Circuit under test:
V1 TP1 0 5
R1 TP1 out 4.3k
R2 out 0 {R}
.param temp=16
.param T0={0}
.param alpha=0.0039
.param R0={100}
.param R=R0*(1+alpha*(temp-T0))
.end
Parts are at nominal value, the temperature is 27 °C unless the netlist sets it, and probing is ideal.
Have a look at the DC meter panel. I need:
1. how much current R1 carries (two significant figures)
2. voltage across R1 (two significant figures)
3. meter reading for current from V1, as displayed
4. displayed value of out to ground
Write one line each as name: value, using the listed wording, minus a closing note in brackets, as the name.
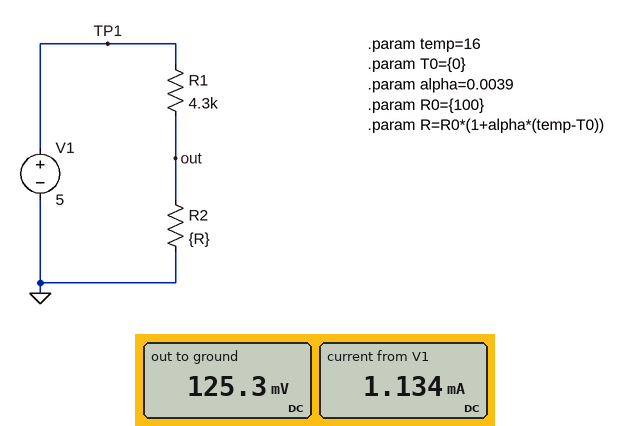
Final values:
how much current R1 carries: 1.1 mA
voltage across R1: 4.9 V
meter reading for current from V1, as displayed: 1.134 mA
displayed value of out to ground: 125.3 mV
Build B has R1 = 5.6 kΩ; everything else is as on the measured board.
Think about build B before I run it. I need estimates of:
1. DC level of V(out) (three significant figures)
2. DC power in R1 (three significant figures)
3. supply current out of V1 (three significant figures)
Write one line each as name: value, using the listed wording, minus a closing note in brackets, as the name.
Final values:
DC level of V(out): 96.8 mV
DC power in R1: 4.29 mW
supply current out of V1: 876 µA
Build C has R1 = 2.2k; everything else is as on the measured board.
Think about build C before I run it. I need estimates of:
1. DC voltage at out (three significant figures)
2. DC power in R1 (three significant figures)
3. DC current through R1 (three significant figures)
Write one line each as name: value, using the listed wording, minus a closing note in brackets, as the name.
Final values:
DC voltage at out: 239 mV
DC power in R1: 10.3 mW
DC current through R1: 2.16 mA
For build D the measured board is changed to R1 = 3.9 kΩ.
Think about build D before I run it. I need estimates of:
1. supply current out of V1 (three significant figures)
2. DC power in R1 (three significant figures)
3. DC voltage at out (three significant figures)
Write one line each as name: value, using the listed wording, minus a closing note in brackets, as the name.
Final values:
supply current out of V1: 1.25 mA
DC power in R1: 6.06 mW
DC voltage at out: 138 mV
